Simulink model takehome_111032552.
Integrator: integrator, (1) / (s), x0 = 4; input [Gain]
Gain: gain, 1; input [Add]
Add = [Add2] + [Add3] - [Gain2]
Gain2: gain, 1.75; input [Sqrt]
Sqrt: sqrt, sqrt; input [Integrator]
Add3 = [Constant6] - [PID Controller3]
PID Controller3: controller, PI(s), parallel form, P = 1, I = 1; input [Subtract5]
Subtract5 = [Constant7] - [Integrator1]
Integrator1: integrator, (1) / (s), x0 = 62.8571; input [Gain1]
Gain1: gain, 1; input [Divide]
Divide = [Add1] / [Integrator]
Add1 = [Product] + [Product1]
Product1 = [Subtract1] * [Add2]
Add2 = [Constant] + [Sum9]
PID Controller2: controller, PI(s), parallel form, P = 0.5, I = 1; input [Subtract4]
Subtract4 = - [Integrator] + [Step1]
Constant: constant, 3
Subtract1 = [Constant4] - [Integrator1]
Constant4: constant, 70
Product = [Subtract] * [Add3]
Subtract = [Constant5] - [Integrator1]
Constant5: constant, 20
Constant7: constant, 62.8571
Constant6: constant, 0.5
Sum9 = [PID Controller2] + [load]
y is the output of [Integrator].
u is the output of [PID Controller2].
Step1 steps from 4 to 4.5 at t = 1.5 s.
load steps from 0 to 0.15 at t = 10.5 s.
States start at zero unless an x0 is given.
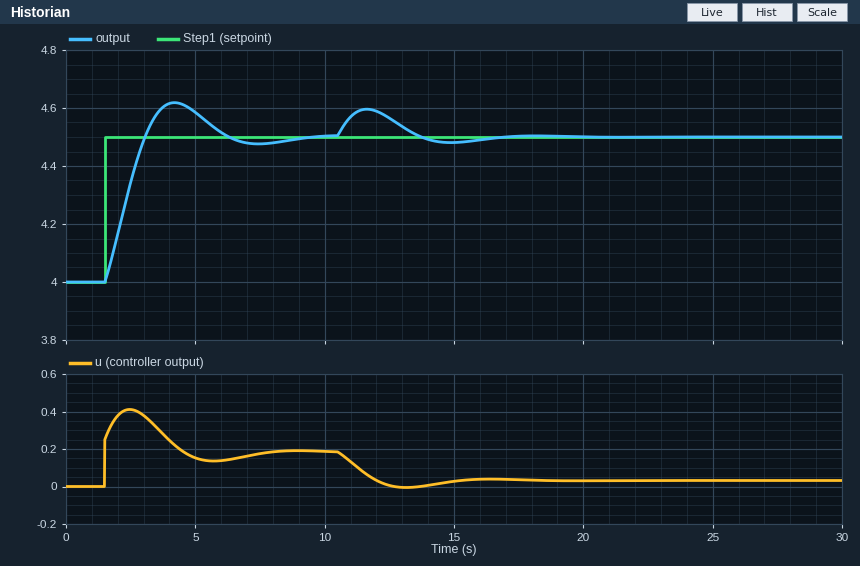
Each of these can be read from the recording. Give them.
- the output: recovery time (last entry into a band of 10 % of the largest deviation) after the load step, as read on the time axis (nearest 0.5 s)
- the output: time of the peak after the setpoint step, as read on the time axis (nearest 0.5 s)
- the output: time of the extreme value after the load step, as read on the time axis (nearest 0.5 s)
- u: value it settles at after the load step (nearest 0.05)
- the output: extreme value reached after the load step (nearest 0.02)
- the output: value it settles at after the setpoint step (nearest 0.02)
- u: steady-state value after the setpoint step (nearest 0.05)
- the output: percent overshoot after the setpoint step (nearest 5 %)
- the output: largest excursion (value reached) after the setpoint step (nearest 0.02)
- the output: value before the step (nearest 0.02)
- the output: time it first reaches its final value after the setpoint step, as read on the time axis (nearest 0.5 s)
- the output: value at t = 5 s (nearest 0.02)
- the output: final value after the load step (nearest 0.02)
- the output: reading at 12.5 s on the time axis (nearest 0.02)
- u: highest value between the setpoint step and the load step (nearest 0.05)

16.0 s
4.0 s
11.5 s
0.05
4.60
4.50
0.20
25 %
4.62
4.00
3.0 s
4.58
4.50
4.56
0.40
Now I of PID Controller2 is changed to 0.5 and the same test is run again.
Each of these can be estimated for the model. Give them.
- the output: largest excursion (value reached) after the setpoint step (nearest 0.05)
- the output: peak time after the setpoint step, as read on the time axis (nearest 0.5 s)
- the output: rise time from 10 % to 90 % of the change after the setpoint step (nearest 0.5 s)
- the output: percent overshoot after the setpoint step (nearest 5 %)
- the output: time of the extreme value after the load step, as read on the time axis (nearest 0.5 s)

4.55
5.5 s
2.0 s
10 %
12.0 s
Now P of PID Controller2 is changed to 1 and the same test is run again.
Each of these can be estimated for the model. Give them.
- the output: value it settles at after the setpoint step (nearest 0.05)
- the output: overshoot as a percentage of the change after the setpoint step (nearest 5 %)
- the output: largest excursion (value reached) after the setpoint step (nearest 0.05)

4.50
10 %
4.55
